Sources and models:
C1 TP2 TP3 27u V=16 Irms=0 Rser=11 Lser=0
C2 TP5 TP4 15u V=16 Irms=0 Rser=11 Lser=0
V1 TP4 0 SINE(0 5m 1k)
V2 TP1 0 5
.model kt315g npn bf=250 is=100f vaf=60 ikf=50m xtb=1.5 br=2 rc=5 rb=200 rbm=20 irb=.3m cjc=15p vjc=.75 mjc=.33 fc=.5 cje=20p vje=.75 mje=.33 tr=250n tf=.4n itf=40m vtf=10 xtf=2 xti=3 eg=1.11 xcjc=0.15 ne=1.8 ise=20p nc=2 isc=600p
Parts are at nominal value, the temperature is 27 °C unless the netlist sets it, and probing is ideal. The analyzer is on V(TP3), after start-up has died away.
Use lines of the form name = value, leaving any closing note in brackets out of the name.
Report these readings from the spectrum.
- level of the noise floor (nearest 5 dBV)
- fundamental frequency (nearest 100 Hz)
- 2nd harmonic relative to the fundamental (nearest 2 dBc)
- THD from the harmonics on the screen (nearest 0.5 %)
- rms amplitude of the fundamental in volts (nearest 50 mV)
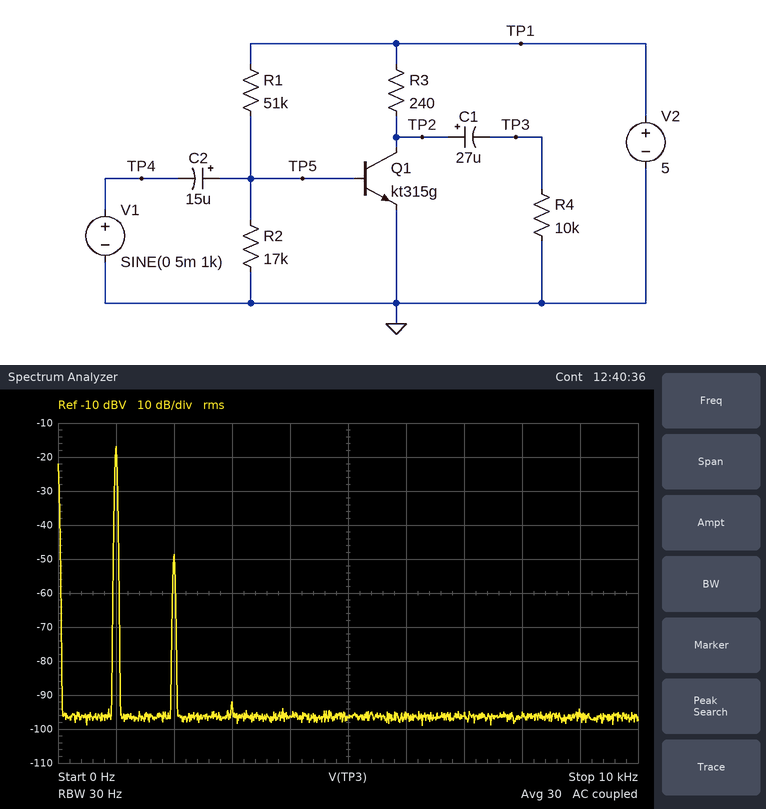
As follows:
level of the noise floor = -95 dBV
fundamental frequency = 1.0 kHz
2nd harmonic relative to the fundamental = -32 dBc
THD from the harmonics on the screen = 2.5 %
rms amplitude of the fundamental in volts = 150 mV
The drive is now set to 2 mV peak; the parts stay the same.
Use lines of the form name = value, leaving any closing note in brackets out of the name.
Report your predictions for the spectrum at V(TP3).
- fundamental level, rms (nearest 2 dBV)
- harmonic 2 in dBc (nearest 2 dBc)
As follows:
fundamental level, rms = -24 dBV
harmonic 2 in dBc = -40 dBc
